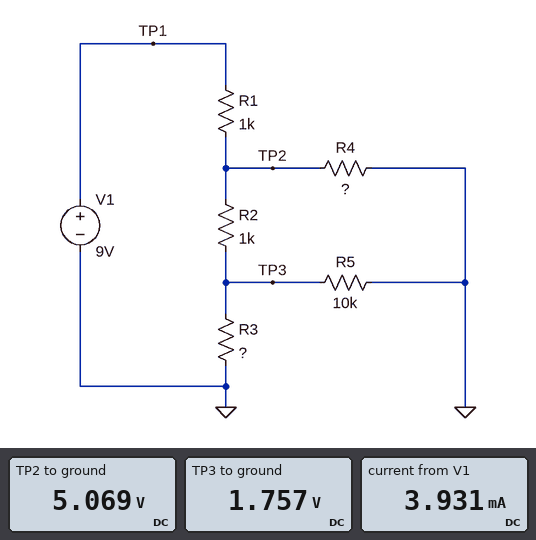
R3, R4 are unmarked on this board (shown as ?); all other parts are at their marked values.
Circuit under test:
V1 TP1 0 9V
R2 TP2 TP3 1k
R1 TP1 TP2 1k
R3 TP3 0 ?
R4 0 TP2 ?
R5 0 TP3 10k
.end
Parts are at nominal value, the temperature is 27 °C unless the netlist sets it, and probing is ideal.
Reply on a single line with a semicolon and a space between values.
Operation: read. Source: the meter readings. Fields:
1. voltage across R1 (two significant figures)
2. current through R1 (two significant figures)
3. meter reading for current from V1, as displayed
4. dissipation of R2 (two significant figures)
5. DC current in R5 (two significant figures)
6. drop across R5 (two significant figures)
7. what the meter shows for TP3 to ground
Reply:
3.9 V; 3.9 mA; 3.931 mA; 11 mW; 180 µA; 1.8 V; 1.757 V
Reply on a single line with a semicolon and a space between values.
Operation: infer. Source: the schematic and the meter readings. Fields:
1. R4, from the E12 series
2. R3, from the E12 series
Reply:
8.2 kΩ; 560 Ω
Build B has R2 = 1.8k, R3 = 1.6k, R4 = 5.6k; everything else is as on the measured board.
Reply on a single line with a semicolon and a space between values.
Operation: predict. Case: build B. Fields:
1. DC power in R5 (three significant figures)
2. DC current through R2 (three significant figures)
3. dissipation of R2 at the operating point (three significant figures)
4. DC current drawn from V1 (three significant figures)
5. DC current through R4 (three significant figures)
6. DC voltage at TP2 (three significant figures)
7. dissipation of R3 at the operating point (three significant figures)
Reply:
684 µW; 1.90 mA; 6.47 mW; 2.97 mA; 1.08 mA; 6.03 V; 4.27 mW
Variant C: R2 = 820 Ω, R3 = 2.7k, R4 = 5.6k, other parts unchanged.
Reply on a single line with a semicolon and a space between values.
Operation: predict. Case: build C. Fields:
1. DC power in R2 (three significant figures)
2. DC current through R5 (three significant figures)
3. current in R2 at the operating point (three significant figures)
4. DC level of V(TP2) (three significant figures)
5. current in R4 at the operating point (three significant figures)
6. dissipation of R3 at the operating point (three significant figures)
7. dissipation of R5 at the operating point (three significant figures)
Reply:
3.32 mW; 428 µA; 2.01 mA; 5.93 V; 1.06 mA; 6.78 mW; 1.83 mW
